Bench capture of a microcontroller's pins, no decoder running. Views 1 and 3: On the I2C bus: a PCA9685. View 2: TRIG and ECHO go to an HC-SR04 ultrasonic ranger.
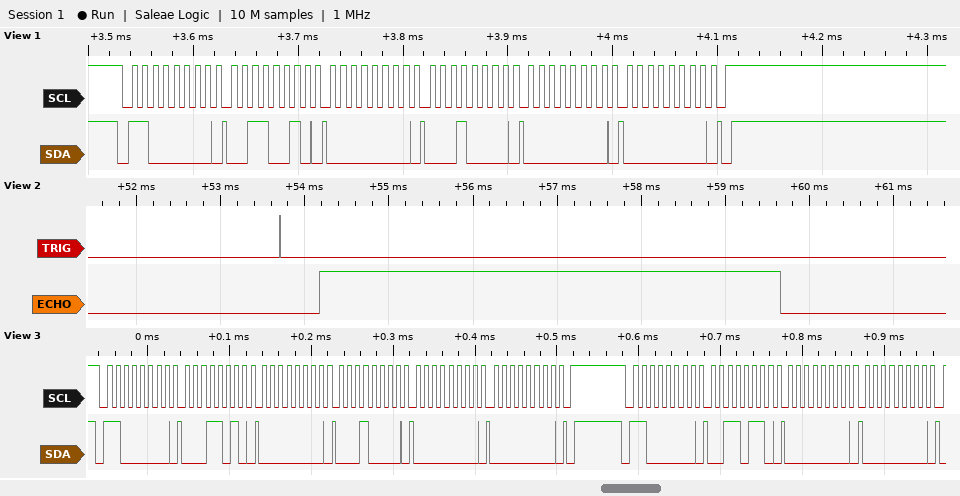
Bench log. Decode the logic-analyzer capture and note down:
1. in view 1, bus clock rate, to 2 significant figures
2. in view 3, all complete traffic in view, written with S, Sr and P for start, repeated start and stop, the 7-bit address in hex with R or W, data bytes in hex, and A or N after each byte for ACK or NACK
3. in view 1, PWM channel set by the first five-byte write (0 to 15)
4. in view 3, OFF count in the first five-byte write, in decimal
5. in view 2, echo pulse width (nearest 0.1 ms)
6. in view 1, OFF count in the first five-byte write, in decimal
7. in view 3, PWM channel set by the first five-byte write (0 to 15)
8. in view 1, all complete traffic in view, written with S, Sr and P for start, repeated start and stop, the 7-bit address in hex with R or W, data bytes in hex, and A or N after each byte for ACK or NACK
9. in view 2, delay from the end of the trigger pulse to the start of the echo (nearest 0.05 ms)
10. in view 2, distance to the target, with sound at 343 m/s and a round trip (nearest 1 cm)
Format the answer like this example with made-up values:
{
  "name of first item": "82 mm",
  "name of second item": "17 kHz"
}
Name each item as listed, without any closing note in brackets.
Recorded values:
{
  "in view 1, bus clock rate, to 2 significant figures": "100 kHz",
  "in view 3, all complete traffic in view, written with S, Sr and P for start, repeated start and stop, the 7-bit address in hex with R or W, data bytes in hex, and A or N after each byte for ACK or NACK": "S 60W A 1A A 00 A 10 A 00 A 00 A P S 60W A 36 A 00 A 00 A",
  "in view 1, PWM channel set by the first five-byte write": "11",
  "in view 3, OFF count in the first five-byte write, in decimal": "0",
  "in view 2, echo pulse width": "5.5 ms",
  "in view 1, OFF count in the first five-byte write, in decimal": "0",
  "in view 3, PWM channel set by the first five-byte write": "5",
  "in view 1, all complete traffic in view, written with S, Sr and P for start, repeated start and stop, the 7-bit address in hex with R or W, data bytes in hex, and A or N after each byte for ACK or NACK": "S 60W A 32 A 00 A 10 A 00 A 00 A P",
  "in view 2, delay from the end of the trigger pulse to the start of the echo": "0.45 ms",
  "in view 2, distance to the target, with sound at 343 m/s and a round trip": "94 cm"
}
